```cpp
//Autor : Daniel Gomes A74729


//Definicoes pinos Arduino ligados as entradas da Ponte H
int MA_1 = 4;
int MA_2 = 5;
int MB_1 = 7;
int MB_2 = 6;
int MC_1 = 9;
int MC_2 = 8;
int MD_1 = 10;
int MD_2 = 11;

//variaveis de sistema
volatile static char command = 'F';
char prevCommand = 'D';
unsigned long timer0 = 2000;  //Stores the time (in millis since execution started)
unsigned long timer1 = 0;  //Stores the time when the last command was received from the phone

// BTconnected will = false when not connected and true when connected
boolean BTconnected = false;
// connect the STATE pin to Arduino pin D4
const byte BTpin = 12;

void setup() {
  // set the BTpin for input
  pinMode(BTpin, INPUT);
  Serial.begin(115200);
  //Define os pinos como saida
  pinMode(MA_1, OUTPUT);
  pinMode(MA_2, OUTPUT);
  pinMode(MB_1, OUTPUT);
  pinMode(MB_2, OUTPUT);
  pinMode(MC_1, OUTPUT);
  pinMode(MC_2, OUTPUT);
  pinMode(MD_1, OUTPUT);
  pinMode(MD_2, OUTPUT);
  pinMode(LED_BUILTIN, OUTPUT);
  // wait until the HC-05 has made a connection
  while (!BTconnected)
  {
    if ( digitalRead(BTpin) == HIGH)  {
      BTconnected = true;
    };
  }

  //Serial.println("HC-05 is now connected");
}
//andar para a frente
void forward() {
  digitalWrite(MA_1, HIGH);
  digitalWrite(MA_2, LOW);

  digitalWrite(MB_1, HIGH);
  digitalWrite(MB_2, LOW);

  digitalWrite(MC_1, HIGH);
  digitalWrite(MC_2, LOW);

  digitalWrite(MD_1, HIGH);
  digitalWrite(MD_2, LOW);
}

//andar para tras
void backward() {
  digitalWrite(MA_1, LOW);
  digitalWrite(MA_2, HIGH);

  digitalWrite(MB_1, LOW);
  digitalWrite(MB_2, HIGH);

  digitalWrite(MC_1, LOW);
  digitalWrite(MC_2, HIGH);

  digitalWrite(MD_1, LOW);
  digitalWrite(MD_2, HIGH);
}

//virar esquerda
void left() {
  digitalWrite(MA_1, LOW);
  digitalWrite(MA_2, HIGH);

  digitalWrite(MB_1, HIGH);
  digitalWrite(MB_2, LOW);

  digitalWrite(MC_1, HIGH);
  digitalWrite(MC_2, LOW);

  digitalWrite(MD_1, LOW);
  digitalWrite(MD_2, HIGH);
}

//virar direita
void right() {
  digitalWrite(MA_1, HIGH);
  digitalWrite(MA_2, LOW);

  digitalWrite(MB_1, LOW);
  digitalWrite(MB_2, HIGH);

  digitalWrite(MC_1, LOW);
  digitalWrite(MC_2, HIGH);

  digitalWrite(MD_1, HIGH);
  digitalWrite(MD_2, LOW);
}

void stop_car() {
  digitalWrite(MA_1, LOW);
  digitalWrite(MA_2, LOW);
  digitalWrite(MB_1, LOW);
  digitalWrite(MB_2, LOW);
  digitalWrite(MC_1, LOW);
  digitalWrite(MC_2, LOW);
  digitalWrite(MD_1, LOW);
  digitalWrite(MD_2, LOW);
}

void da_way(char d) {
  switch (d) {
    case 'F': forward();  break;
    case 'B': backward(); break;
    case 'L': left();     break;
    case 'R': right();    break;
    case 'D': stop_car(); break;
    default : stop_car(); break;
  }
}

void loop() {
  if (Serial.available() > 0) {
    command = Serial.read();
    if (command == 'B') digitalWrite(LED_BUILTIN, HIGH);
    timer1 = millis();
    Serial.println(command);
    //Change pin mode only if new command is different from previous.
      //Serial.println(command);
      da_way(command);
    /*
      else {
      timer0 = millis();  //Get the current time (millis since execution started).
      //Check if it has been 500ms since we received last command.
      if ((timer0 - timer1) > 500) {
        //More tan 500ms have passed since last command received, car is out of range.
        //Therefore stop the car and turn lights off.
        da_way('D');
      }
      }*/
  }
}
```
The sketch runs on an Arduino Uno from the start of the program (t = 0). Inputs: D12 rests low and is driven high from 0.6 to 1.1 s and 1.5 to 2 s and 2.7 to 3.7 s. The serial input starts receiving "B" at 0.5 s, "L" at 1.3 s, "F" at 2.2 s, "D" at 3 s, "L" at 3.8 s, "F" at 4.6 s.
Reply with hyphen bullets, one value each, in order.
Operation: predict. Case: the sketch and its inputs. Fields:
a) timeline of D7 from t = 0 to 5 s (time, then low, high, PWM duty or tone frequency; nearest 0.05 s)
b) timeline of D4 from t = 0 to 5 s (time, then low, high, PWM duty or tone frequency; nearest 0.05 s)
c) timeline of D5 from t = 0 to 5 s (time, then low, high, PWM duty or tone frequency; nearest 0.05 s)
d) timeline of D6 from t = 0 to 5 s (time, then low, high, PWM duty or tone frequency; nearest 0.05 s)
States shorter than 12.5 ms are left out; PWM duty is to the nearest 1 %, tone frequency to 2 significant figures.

- 0 s low; 1.3 s high; 3 s low; 3.8 s high
- 0 s low; 2.2 s high; 3 s low; 4.6 s high
- 0 s low; 0.6 s high; 2.2 s low; 3.8 s high; 4.6 s low
- 0 s low; 0.6 s high; 1.3 s low
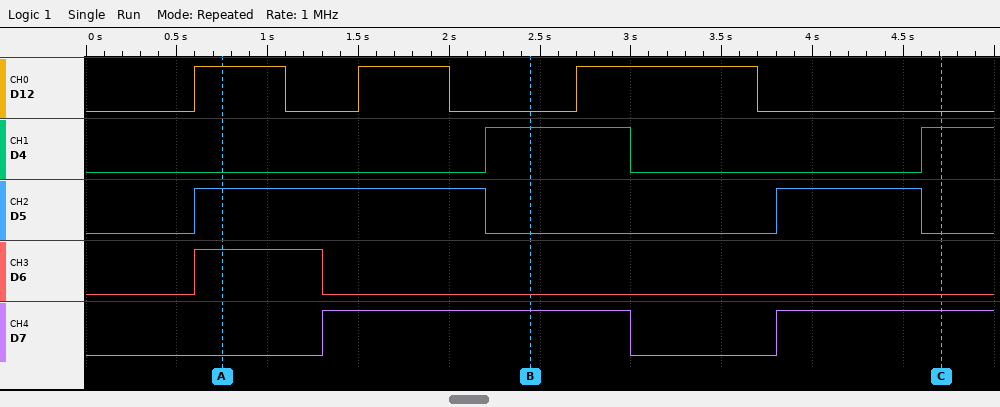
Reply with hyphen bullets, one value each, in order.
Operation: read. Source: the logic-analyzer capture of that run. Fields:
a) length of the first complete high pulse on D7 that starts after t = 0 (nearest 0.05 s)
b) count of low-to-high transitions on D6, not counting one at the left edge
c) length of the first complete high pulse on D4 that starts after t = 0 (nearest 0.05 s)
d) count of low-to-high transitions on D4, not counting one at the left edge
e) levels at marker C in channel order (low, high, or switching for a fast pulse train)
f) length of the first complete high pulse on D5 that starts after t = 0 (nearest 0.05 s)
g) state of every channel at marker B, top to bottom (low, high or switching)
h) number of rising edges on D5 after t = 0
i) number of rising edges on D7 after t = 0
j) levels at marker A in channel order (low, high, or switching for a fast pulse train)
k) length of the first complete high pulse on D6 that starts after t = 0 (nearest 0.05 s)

- 1.70 s
- 1
- 0.80 s
- 2
- D12 low, D4 high, D5 low, D6 low, D7 high
- 1.60 s
- D12 low, D4 high, D5 low, D6 low, D7 high
- 2
- 2
- D12 high, D4 low, D5 high, D6 high, D7 low
- 0.70 s
